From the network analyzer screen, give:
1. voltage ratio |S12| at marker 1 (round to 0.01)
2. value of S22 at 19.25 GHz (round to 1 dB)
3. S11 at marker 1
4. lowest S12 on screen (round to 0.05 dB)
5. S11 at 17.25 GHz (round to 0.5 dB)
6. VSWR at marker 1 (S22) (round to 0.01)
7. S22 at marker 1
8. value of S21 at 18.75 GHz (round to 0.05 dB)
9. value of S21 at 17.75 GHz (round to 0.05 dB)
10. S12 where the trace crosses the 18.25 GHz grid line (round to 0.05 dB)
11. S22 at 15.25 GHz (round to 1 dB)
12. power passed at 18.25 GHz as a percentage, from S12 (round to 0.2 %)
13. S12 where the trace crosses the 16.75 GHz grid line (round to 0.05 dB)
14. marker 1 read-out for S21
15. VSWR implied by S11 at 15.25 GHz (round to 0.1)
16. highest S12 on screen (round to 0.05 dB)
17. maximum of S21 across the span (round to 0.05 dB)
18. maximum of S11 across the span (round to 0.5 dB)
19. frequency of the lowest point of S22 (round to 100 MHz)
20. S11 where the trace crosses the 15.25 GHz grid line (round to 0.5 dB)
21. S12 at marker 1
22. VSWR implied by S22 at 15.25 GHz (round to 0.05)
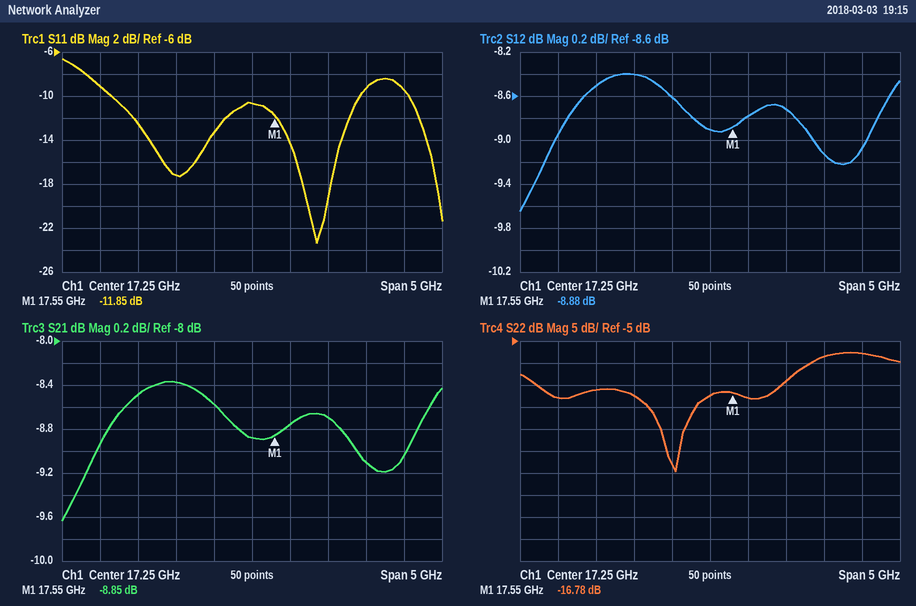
0.36
-8 dB
-11.85 dB
-9.65 dB
-10.5 dB
1.34
-16.78 dB
-9.10 dB
-8.75 dB
-8.70 dB
-18 dB
13.4 %
-8.60 dB
-8.85 dB
2.1
-8.40 dB
-8.35 dB
-6.5 dB
16.8 GHz
-9.0 dB
-8.88 dB
1.30
